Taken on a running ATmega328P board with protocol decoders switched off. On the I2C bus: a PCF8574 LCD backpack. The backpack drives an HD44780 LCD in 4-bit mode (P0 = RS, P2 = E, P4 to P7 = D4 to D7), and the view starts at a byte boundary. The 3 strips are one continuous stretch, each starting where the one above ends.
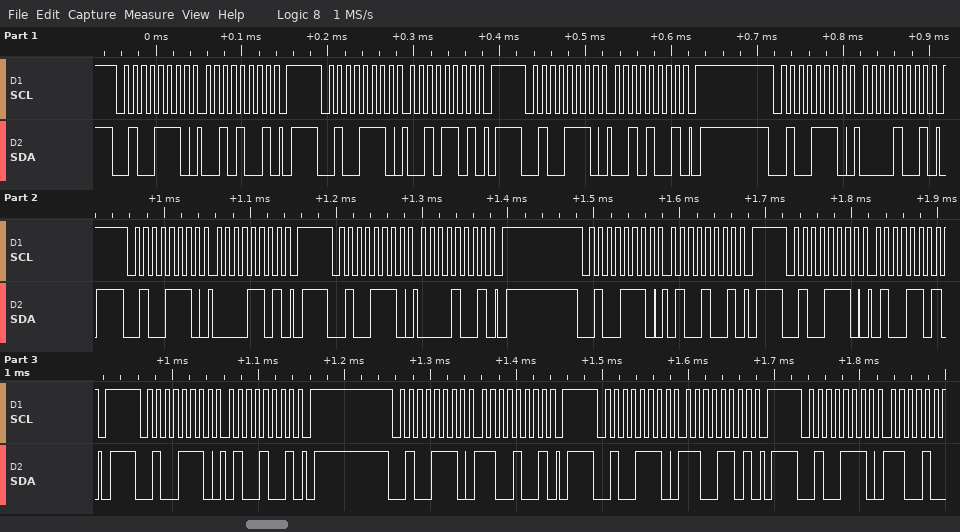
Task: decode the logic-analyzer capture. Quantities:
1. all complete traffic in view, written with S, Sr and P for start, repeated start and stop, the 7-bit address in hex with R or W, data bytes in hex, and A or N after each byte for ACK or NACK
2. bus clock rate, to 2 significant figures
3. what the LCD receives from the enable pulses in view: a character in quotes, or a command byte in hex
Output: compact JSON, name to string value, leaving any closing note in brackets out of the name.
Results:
{"all complete traffic in view, written with S, Sr and P for start, repeated start and stop, the 7-bit address in hex with R or W, data bytes in hex, and A or N after each byte for ACK or NACK": "S 27W A 29 A P S 27W A 2D A P S 27W A 29 A P S 27W A 09 A P S 27W A 0D A P S 27W A 09 A P S 27W A 49 A P S 27W A 4D A P S 27W A 49 A P S 27W A C9 A P S 27W A CD A P S 27W A", "bus clock rate, to 2 significant figures": "100 kHz", "what the LCD receives from the enable pulses in view: a character in quotes, or a command byte in hex": "' '"}
